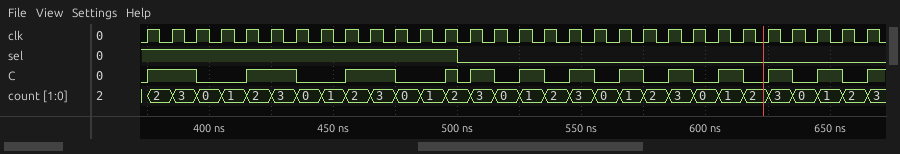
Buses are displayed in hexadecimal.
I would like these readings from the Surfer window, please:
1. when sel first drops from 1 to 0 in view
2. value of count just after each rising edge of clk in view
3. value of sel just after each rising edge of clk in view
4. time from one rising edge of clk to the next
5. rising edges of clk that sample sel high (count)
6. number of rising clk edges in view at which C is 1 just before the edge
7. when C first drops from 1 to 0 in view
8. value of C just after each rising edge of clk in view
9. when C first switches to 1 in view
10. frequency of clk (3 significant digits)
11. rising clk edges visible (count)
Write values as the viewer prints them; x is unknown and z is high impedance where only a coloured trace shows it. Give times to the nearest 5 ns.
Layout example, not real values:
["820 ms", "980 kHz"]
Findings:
["500 ns", "2, 3, 0, 1, 2, 3, 0, 1, 2, 3, 0, 1, 2, 3, 0, 1, 2, 3, 0, 1, 2, 3, 0, 1, 2, 3, 0, 1, 2, 3", "1 1 1 1 1 1 1 1 1 1 1 1 1 0 0 0 0 0 0 0 0 0 0 0 0 0 0 0 0 0", "10 ns", "13", "14", "395 ns", "1 1 0 0 1 1 0 0 1 1 0 0 1 1 0 1 0 1 0 1 0 1 0 1 0 1 0 1 0 1", "375 ns", "100 MHz", "30"]
